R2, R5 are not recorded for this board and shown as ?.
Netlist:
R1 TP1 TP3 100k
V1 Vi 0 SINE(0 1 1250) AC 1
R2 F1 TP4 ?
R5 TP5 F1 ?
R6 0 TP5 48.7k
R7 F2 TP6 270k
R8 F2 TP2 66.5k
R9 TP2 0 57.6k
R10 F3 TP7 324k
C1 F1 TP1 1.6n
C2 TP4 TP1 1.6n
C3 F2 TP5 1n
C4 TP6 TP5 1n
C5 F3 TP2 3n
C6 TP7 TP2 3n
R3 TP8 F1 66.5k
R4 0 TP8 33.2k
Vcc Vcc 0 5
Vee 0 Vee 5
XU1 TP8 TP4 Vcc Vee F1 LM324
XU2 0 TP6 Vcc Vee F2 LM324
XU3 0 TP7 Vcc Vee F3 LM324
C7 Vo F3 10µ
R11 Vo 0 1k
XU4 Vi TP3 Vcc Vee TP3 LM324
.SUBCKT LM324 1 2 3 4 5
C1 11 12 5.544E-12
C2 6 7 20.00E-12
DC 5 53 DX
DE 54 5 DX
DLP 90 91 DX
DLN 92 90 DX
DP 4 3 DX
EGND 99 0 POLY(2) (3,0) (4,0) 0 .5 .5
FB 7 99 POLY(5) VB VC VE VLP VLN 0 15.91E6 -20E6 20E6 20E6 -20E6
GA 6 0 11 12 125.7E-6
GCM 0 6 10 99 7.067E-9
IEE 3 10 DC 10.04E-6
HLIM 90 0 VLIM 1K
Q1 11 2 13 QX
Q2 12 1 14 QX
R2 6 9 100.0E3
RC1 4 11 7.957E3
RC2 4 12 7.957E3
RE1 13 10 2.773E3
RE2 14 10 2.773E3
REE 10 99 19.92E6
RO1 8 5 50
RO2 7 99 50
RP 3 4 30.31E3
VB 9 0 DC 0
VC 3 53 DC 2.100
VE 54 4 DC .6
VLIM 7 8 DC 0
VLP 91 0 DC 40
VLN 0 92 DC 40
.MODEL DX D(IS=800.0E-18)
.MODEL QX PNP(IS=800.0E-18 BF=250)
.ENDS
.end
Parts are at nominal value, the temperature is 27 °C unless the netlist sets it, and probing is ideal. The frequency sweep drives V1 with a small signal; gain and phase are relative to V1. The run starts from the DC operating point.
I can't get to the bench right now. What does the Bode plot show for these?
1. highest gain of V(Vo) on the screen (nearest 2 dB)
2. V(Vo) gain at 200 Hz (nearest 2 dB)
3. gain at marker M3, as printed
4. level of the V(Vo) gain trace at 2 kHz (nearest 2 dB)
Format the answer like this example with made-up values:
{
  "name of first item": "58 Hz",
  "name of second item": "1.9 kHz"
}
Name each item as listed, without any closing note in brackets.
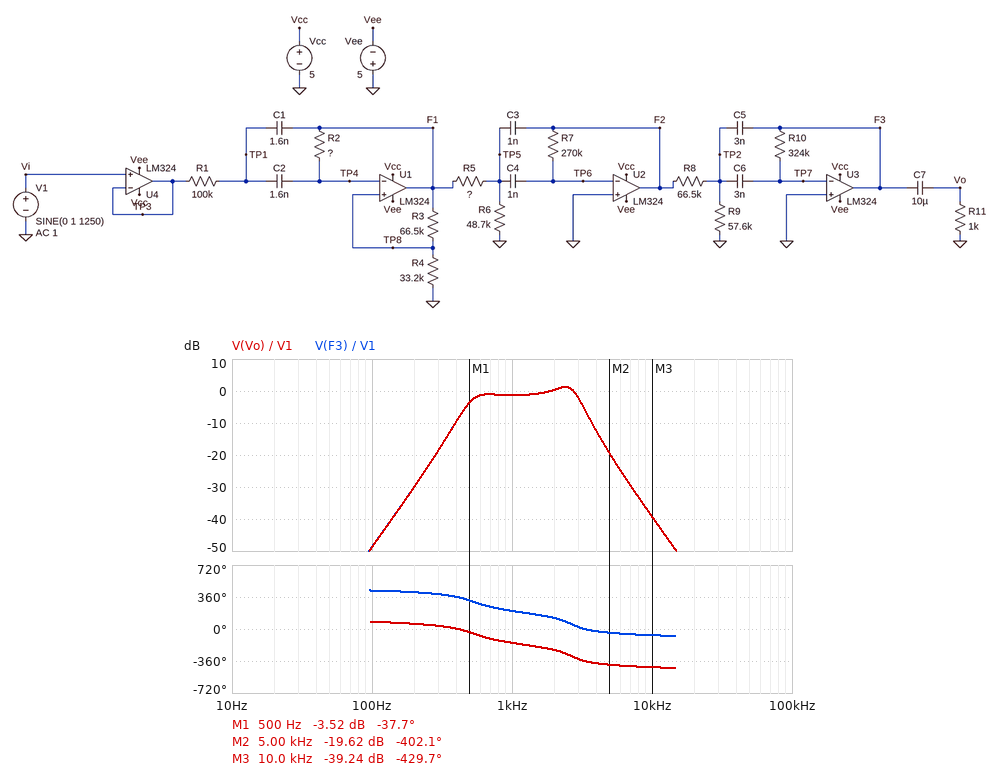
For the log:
{
  "highest gain of V(Vo) on the screen": "2 dB",
  "V(Vo) gain at 200 Hz": "-30 dB",
  "gain at marker M3, as printed": "-39.24 dB",
  "level of the V(Vo) gain trace at 2 kHz": "0 dB"
}
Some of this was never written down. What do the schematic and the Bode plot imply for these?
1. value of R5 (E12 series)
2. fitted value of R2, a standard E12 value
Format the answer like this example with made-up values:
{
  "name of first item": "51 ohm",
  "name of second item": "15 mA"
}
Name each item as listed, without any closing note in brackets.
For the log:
{
  "value of R5": "18 kΩ",
  "fitted value of R2, a standard E12 value": "68 kΩ"
}
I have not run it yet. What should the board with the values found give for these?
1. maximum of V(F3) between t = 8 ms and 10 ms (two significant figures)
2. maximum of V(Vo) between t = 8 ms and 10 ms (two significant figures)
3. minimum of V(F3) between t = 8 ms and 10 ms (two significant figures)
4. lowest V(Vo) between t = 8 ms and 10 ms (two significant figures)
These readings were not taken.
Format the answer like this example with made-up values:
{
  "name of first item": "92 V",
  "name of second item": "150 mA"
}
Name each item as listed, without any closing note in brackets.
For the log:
{
  "maximum of V(F3) between t = 8 ms and 10 ms": "870 mV",
  "maximum of V(Vo) between t = 8 ms and 10 ms": "870 mV",
  "minimum of V(F3) between t = 8 ms and 10 ms": "-880 mV",
  "lowest V(Vo) between t = 8 ms and 10 ms": "-870 mV"
}
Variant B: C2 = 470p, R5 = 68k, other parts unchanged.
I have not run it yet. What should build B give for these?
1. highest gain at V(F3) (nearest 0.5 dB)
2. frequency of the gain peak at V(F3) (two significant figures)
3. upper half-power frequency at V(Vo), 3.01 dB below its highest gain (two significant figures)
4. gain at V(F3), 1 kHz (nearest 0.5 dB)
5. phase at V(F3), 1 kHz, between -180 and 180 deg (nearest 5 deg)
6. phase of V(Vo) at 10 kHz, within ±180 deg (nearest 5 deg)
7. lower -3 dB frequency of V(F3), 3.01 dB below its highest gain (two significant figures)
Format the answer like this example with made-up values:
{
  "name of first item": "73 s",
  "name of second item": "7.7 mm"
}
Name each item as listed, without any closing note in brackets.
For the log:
{
  "highest gain at V(F3)": "-12.0 dB",
  "frequency of the gain peak at V(F3)": "1.6 kHz",
  "upper half-power frequency at V(Vo), 3.01 dB below its highest gain": "2.1 kHz",
  "gain at V(F3), 1 kHz": "-14.5 dB",
  "phase at V(F3), 1 kHz, between -180 and 180 deg": "-150 deg",
  "phase of V(Vo) at 10 kHz, within ±180 deg": "-50 deg",
  "lower -3 dB frequency of V(F3), 3.01 dB below its highest gain": "730 Hz"
}
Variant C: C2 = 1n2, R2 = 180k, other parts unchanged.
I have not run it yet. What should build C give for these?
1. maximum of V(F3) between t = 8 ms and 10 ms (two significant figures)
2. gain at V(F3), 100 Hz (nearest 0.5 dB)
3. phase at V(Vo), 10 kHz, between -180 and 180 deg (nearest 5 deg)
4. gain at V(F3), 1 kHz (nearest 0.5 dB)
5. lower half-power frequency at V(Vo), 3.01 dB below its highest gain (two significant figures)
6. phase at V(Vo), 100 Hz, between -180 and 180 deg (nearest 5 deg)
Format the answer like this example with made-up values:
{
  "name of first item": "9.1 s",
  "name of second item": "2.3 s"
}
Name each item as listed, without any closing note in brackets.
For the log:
{
  "maximum of V(F3) between t = 8 ms and 10 ms": "2.0 V",
  "gain at V(F3), 100 Hz": "-42.5 dB",
  "phase at V(Vo), 10 kHz, between -180 and 180 deg": "-80 deg",
  "gain at V(F3), 1 kHz": "8.0 dB",
  "lower half-power frequency at V(Vo), 3.01 dB below its highest gain": "520 Hz",
  "phase at V(Vo), 100 Hz, between -180 and 180 deg": "85 deg"
}
